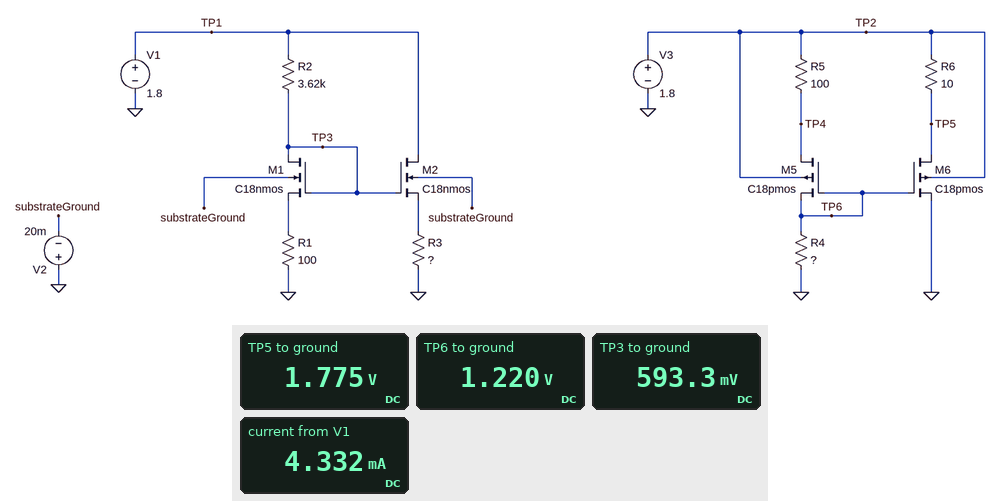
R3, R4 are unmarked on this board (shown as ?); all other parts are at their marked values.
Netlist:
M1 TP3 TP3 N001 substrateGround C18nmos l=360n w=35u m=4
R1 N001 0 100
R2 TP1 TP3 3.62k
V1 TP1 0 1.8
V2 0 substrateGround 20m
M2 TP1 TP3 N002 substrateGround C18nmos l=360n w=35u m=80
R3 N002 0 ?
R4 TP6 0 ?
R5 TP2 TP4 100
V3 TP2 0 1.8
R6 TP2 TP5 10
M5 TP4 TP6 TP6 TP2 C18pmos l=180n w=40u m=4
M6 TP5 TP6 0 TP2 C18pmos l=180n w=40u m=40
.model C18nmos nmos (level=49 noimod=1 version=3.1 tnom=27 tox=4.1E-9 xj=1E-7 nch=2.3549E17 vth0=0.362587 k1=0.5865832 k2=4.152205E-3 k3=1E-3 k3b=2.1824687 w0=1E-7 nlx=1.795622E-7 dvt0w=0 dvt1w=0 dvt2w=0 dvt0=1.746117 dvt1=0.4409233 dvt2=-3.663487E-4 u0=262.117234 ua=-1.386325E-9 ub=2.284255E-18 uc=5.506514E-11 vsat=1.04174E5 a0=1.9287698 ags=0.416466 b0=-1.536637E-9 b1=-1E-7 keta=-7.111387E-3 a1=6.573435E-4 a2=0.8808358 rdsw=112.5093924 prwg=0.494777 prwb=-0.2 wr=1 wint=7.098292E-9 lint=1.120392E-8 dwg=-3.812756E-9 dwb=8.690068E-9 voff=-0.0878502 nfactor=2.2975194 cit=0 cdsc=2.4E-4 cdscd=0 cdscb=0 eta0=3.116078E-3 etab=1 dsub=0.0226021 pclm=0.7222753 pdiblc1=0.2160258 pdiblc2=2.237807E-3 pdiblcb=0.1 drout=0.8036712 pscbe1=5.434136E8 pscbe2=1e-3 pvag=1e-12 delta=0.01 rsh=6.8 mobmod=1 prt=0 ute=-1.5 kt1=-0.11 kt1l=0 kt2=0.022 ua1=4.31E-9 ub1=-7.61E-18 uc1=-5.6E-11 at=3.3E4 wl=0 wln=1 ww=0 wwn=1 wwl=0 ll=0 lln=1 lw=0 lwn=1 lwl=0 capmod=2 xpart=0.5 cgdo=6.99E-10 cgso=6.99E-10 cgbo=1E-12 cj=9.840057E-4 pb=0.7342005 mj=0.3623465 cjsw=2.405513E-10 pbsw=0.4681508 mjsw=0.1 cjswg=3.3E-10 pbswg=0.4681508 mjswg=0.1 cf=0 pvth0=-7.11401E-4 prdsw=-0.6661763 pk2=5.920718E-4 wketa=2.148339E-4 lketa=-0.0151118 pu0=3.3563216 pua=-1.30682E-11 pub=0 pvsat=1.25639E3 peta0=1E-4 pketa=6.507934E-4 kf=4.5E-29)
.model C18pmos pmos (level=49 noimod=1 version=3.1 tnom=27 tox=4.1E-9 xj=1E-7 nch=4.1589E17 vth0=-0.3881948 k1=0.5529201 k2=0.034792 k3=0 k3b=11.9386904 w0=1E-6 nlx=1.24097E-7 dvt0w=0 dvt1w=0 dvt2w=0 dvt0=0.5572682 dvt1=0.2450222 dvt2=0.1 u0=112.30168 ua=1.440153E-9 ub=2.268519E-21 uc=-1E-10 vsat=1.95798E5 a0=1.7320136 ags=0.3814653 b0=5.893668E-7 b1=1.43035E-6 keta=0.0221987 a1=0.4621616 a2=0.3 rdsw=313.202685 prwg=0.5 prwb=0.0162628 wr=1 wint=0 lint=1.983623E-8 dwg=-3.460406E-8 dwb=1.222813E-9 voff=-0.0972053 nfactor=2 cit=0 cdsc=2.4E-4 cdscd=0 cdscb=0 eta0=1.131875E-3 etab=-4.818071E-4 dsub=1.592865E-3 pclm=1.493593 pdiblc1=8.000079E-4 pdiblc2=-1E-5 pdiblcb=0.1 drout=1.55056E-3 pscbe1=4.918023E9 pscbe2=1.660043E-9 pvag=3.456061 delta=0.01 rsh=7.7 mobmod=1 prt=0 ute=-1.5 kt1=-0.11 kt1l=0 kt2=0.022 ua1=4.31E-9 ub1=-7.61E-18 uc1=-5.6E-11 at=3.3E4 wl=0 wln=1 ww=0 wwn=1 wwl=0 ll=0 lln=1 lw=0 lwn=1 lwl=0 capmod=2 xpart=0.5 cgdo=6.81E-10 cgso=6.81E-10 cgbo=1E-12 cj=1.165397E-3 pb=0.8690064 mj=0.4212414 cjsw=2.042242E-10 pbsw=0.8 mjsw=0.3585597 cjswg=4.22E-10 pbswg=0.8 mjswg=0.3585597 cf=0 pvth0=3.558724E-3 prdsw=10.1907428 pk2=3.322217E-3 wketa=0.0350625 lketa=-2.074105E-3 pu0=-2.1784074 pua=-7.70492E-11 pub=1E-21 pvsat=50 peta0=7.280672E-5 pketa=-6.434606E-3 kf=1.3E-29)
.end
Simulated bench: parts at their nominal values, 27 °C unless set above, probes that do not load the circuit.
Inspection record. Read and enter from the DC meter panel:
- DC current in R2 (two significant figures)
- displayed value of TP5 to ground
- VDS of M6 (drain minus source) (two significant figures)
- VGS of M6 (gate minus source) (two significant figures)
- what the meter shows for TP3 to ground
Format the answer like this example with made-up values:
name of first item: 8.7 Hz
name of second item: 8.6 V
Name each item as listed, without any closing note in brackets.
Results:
DC current in R2: 330 µA
displayed value of TP5 to ground: 1.775 V
VDS of M6 (drain minus source): 1.8 V
VGS of M6 (gate minus source): 1.2 V
what the meter shows for TP3 to ground: 593.3 mV
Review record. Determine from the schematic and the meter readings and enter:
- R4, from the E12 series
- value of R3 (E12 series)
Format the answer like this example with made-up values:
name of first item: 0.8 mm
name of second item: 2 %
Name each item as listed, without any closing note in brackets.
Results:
R4, from the E12 series: 5.6 kΩ
value of R3: 15 Ω
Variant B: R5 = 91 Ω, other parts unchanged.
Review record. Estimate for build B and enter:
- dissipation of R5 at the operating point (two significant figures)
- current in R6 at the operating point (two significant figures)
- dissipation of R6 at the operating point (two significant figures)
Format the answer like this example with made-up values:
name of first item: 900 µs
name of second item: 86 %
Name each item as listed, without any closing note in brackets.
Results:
dissipation of R5 at the operating point: 4.3 µW
current in R6 at the operating point: 2.4 mA
dissipation of R6 at the operating point: 57 µW
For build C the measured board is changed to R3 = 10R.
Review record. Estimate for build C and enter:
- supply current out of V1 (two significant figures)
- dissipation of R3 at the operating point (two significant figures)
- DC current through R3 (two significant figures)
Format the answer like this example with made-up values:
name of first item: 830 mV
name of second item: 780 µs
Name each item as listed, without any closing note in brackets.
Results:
supply current out of V1: 5.4 mA
dissipation of R3 at the operating point: 260 µW
DC current through R3: 5.1 mA
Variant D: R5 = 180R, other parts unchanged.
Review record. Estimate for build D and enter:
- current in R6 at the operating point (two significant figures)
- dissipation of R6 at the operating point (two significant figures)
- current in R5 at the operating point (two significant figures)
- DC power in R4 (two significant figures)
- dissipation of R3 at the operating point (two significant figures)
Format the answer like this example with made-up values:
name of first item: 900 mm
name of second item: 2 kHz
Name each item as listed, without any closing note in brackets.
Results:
current in R6 at the operating point: 3.1 mA
dissipation of R6 at the operating point: 94 µW
current in R5 at the operating point: 210 µA
DC power in R4: 260 µW
dissipation of R3 at the operating point: 240 µW
